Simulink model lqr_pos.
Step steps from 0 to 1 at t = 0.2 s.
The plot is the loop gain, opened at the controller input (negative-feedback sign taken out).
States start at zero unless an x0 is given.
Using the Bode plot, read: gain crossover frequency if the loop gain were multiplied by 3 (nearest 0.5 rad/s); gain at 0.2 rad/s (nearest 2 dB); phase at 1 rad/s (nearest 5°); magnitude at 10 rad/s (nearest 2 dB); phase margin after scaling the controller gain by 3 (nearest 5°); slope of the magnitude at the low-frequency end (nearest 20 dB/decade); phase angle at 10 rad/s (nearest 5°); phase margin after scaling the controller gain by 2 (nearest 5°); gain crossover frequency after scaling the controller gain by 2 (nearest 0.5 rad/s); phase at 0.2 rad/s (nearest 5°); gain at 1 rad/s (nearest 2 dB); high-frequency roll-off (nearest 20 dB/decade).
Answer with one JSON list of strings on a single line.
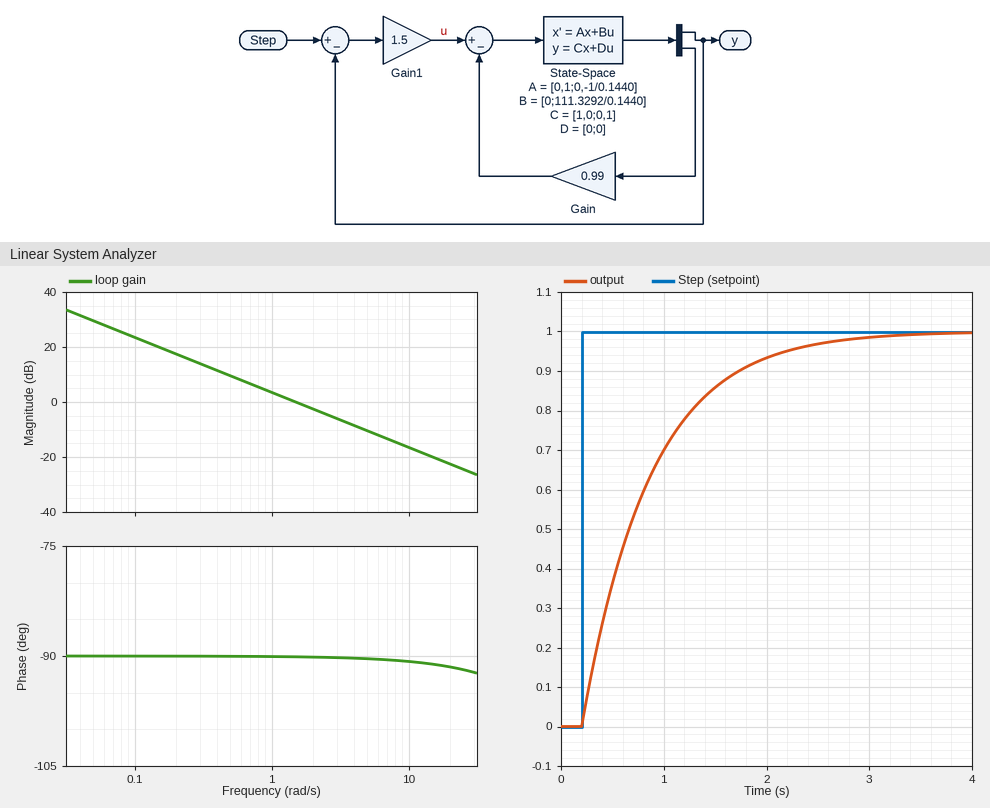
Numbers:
["4.5 rad/s", "18 dB", "-90°", "-16 dB", "90°", "-20 dB/decade", "-90°", "90°", "3.0 rad/s", "-90°", "4 dB", "-20 dB/decade"]
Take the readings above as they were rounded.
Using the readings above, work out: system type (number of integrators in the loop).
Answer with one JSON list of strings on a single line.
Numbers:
["1"]
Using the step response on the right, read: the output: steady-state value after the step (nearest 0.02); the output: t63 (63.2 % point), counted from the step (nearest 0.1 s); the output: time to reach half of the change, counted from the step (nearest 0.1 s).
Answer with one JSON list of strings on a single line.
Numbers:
["1.00", "0.7 s", "0.5 s"]
